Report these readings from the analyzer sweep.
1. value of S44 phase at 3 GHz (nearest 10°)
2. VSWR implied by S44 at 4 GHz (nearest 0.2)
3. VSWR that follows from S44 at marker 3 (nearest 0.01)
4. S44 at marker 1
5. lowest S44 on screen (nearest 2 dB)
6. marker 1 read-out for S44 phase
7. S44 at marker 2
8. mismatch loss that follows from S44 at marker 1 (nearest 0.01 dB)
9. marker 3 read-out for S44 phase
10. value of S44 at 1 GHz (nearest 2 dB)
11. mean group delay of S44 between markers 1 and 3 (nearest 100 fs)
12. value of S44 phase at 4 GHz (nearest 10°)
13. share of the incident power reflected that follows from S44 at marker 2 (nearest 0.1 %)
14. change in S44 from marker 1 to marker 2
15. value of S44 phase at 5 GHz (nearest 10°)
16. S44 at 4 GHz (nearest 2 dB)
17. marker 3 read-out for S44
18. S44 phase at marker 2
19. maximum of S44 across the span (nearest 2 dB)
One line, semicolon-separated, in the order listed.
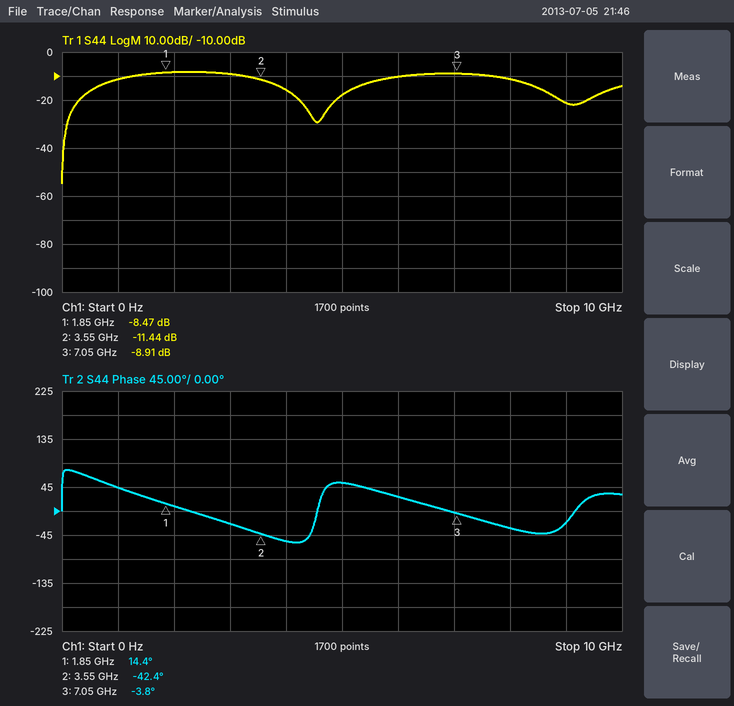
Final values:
-20°; 1.4; 2.12; -8.47 dB; -54 dB; 14.4°; -11.44 dB; 0.67 dB; -3.8°; -12 dB; 9.7 ps; -60°; 7.2 %; -2.97 dB; 50°; -16 dB; -8.91 dB; -42.4°; -8 dB
